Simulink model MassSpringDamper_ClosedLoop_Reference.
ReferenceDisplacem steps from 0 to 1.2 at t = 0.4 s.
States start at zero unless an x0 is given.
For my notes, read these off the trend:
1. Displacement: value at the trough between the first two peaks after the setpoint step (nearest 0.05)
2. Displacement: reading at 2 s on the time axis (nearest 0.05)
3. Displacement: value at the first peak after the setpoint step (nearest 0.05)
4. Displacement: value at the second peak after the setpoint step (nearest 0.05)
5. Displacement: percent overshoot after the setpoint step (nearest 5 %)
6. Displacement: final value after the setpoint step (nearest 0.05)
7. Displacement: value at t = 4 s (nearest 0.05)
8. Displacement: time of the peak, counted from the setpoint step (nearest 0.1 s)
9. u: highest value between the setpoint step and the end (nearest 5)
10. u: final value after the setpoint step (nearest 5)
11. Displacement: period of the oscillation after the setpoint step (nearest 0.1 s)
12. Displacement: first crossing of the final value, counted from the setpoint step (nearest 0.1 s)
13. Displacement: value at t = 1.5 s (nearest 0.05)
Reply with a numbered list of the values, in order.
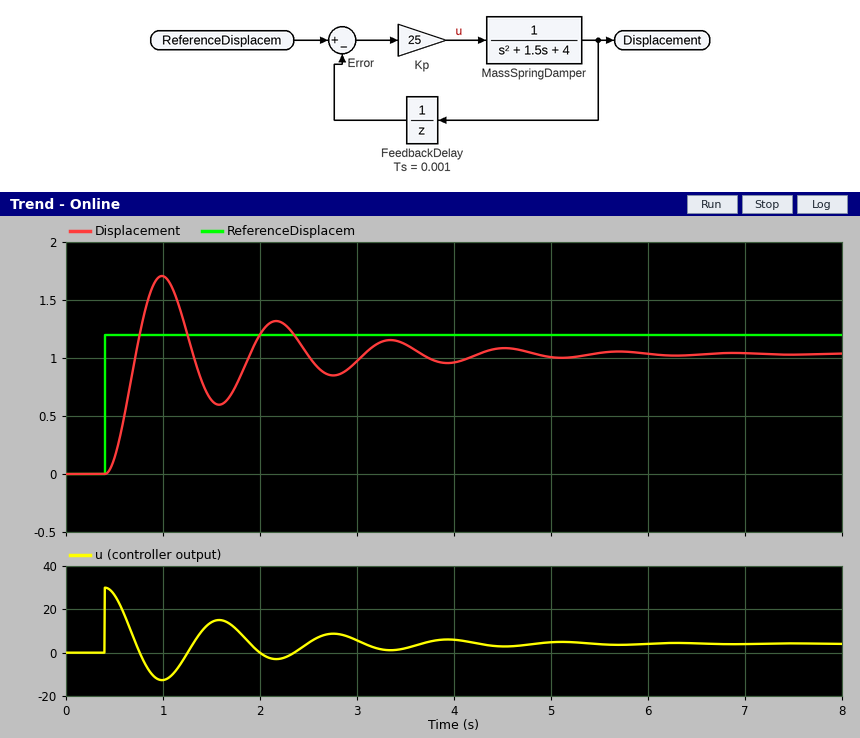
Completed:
1. 0.60
2. 1.20
3. 1.70
4. 1.30
5. 65 %
6. 1.05
7. 0.95
8. 0.6 s
9. 30
10. 5
11. 1.2 s
12. 0.3 s
13. 0.65
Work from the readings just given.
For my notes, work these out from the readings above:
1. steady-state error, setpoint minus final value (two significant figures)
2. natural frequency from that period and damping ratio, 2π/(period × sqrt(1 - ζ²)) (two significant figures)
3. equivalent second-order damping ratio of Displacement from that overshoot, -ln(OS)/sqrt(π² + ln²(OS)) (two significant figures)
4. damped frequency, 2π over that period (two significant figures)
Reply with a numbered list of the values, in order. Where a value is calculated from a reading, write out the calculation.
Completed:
1. 1.2 - 1.05 = 0.15
2. 2π / (1.2 × sqrt(1 - 0.14²)) = 5.3 rad/s
3. ln(0.65) = -0.431; 0.431 / sqrt(9.870 + 0.186) = 0.14
4. 2π / 1.2 = 5.2 rad/s
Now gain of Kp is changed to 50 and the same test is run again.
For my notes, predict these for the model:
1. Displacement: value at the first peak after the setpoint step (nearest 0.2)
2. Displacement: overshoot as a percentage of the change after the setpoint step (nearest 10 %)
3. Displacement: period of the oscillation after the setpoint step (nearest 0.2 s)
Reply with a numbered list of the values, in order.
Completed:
1. 2.0
2. 70 %
3. 0.8 s
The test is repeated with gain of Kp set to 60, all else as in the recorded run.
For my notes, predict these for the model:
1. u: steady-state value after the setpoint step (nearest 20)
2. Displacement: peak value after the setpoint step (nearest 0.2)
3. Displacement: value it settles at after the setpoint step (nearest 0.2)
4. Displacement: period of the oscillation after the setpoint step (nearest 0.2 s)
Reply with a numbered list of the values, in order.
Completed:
1. 0
2. 2.0
3. 1.2
4. 0.8 s
